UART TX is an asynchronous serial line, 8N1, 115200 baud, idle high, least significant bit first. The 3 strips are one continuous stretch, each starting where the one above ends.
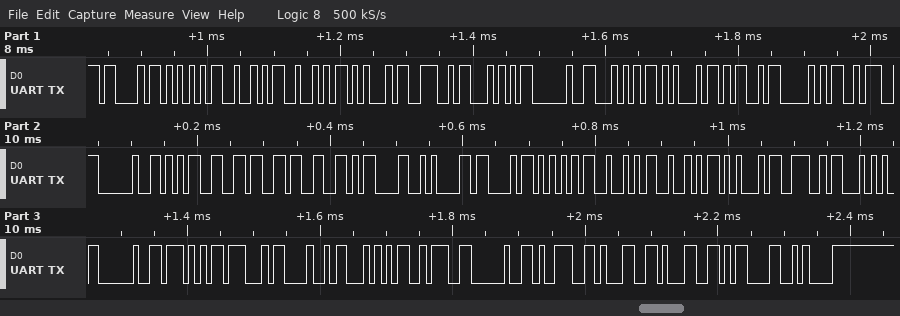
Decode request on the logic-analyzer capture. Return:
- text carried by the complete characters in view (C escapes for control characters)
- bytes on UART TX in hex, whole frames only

"CURRENT TEMP: 563\r\nCURRENT WGHT: 911\r\n"
0x43 0x55 0x52 0x52 0x45 0x4E 0x54 0x20 0x54 0x45 0x4D 0x50 0x3A 0x20 0x35 0x36 0x33 0x0D 0x0A 0x43 0x55 0x52 0x52 0x45 0x4E 0x54 0x20 0x57 0x47 0x48 0x54 0x3A 0x20 0x39 0x31 0x31 0x0D 0x0A
